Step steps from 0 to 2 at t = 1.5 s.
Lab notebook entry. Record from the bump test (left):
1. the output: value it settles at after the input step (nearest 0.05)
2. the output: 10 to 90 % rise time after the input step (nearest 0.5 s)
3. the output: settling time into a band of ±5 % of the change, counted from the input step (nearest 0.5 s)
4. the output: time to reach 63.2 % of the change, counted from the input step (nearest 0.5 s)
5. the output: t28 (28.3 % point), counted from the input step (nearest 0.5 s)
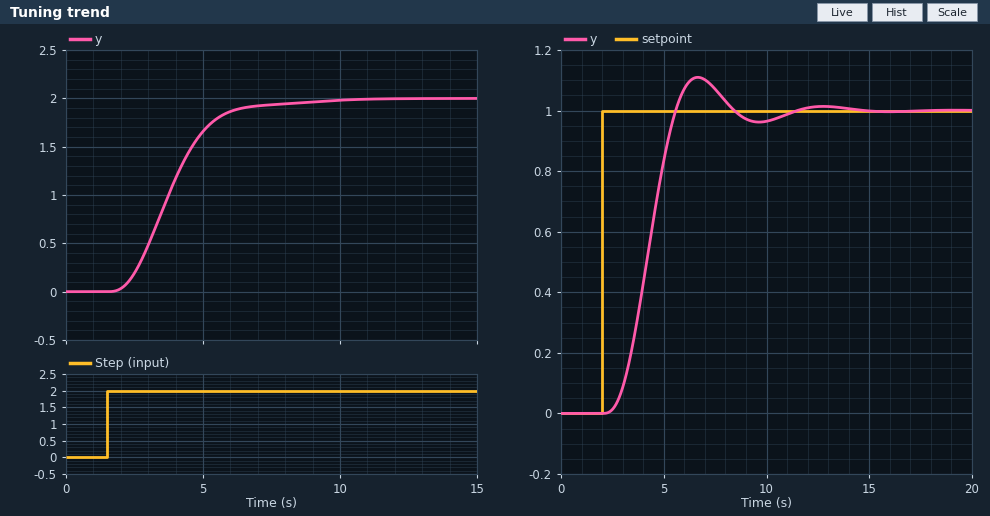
2.00
3.0 s
5.0 s
2.5 s
1.5 s
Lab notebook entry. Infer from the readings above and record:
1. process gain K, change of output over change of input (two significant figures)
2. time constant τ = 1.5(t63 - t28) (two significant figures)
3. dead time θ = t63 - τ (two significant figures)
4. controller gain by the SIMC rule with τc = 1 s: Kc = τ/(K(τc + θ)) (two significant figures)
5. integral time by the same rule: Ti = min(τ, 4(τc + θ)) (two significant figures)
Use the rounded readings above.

1.0
1.5 s
1.0 s
0.75
1.5 s
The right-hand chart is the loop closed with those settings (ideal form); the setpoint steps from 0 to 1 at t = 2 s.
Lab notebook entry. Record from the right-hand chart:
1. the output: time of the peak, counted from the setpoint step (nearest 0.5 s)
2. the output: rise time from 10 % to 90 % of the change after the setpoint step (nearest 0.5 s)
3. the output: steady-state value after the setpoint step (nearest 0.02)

4.5 s
2.0 s
1.00
